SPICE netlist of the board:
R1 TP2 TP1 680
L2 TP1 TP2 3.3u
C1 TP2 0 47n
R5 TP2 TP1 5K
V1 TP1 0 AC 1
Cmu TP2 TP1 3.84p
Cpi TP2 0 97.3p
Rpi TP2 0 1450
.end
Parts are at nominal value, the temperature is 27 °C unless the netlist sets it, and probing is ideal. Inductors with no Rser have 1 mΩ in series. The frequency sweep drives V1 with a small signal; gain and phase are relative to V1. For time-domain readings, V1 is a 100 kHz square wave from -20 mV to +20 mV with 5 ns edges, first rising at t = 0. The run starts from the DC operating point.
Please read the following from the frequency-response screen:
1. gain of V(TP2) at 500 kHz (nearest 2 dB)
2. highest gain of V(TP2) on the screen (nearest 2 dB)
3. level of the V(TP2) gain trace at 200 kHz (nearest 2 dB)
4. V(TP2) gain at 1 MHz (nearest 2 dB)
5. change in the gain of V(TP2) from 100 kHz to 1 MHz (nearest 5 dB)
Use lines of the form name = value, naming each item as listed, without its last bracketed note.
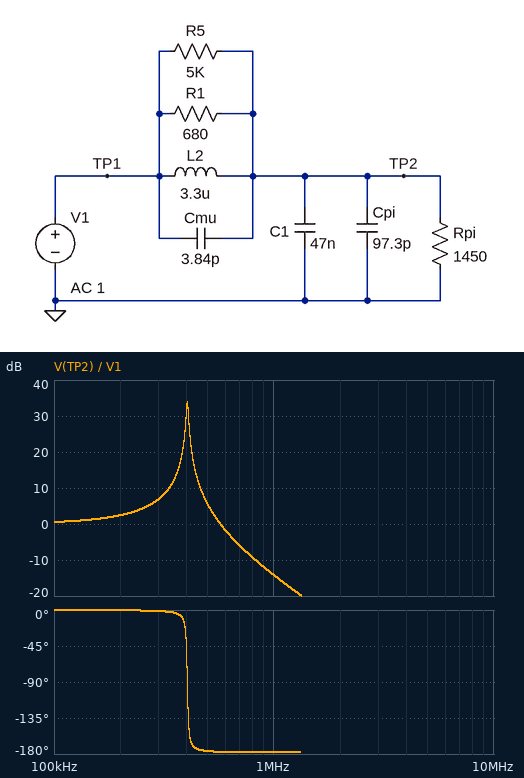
gain of V(TP2) at 500 kHz = 6 dB
highest gain of V(TP2) on the screen = 34 dB
level of the V(TP2) gain trace at 200 kHz = 2 dB
V(TP2) gain at 1 MHz = -14 dB
change in the gain of V(TP2) from 100 kHz to 1 MHz = -15 dB
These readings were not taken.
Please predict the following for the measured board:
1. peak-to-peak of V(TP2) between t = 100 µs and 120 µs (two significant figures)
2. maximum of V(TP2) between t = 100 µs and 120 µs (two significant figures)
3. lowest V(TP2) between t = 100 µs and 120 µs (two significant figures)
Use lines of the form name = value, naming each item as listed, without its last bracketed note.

peak-to-peak of V(TP2) between t = 100 µs and 120 µs = 81 mV
maximum of V(TP2) between t = 100 µs and 120 µs = 40 mV
lowest V(TP2) between t = 100 µs and 120 µs = -42 mV
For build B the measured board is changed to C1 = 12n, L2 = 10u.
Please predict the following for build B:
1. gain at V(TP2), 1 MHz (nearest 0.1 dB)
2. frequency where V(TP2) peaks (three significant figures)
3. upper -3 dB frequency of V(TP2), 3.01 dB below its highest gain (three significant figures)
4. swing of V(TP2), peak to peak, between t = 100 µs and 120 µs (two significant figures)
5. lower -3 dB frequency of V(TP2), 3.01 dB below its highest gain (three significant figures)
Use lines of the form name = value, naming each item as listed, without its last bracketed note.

gain at V(TP2), 1 MHz = -11.5 dB
frequency where V(TP2) peaks = 457 kHz
upper -3 dB frequency of V(TP2), 3.01 dB below its highest gain = 472 kHz
swing of V(TP2), peak to peak, between t = 100 µs and 120 µs = 110 mV
lower -3 dB frequency of V(TP2), 3.01 dB below its highest gain = 441 kHz
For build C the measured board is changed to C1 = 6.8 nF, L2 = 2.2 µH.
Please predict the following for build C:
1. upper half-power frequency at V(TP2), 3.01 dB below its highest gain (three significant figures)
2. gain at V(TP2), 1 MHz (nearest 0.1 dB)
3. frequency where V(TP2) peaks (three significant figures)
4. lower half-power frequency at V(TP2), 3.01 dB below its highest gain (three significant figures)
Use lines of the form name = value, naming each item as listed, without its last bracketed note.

upper half-power frequency at V(TP2), 3.01 dB below its highest gain = 1.32 MHz
gain at V(TP2), 1 MHz = 7.9 dB
frequency where V(TP2) peaks = 1.29 MHz
lower half-power frequency at V(TP2), 3.01 dB below its highest gain = 1.26 MHz
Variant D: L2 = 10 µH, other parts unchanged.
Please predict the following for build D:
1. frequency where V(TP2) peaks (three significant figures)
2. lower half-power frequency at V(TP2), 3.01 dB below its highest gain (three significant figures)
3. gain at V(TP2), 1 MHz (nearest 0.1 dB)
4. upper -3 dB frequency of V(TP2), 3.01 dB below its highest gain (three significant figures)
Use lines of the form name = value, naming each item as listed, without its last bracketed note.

frequency where V(TP2) peaks = 232 kHz
lower half-power frequency at V(TP2), 3.01 dB below its highest gain = 228 kHz
gain at V(TP2), 1 MHz = -24.9 dB
upper -3 dB frequency of V(TP2), 3.01 dB below its highest gain = 236 kHz
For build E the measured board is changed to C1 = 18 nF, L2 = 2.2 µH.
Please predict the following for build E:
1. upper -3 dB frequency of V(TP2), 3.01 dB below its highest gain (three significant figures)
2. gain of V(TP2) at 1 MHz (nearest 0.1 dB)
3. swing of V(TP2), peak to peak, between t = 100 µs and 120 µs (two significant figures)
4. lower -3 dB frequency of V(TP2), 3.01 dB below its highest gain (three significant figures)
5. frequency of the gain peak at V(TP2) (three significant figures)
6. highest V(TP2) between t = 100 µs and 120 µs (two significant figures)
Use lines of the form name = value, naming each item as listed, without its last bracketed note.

upper -3 dB frequency of V(TP2), 3.01 dB below its highest gain = 808 kHz
gain of V(TP2) at 1 MHz = 4.8 dB
swing of V(TP2), peak to peak, between t = 100 µs and 120 µs = 85 mV
lower -3 dB frequency of V(TP2), 3.01 dB below its highest gain = 787 kHz
frequency of the gain peak at V(TP2) = 797 kHz
highest V(TP2) between t = 100 µs and 120 µs = 42 mV
